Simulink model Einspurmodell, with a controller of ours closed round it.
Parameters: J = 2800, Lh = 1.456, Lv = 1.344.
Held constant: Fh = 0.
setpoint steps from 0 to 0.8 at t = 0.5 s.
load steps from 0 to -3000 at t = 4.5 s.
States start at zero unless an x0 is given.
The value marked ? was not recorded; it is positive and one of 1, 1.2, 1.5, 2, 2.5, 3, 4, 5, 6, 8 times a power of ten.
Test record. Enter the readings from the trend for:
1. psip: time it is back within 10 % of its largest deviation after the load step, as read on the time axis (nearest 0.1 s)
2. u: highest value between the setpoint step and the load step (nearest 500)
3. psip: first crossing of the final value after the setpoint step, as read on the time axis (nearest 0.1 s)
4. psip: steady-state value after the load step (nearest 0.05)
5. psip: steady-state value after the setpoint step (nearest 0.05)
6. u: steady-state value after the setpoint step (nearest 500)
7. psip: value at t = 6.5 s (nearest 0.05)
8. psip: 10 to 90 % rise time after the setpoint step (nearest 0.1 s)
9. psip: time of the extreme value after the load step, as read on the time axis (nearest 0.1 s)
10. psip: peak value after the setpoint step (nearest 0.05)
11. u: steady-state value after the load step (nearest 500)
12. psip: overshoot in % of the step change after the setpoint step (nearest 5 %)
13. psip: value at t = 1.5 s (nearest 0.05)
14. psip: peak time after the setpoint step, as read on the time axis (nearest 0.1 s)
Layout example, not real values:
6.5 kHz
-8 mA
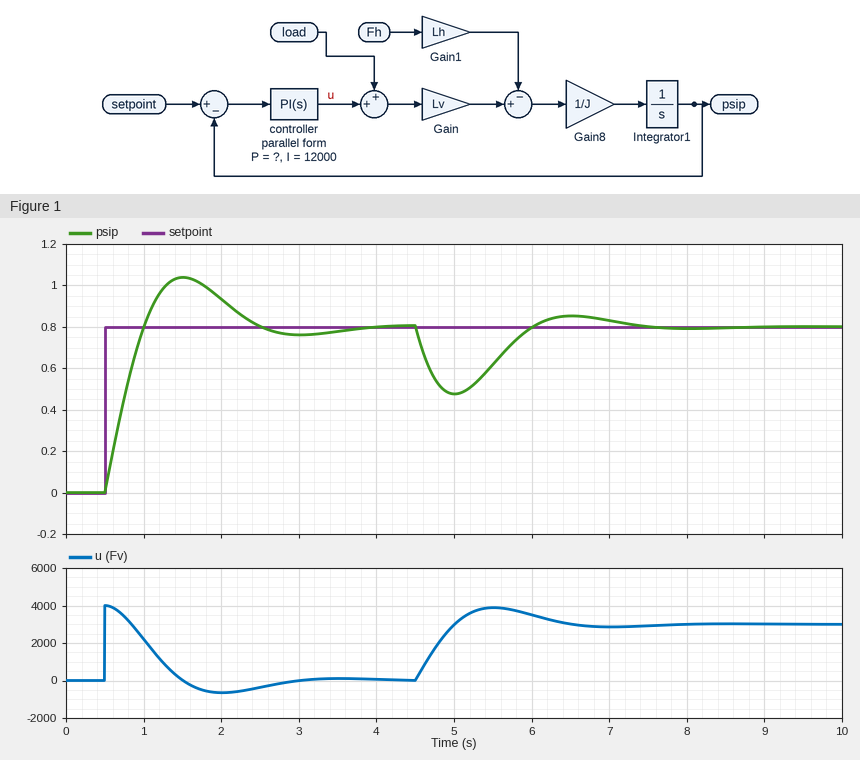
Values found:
7.0 s
4000
1.0 s
0.80
0.80
0
0.85
0.4 s
5.0 s
1.05
3000
30 %
1.05
1.5 s
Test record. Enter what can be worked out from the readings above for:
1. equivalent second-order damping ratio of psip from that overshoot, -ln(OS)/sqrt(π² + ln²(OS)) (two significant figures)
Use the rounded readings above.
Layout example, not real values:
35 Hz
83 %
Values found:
0.36
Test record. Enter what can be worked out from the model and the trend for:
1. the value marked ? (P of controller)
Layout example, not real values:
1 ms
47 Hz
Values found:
5000
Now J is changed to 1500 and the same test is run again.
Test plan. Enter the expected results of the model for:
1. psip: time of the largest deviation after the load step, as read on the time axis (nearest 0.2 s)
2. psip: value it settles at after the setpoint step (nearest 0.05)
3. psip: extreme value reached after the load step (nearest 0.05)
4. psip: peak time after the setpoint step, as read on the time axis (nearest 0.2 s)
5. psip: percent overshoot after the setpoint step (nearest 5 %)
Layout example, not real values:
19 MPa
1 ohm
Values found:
4.8 s
0.80
0.40
1.2 s
20 %
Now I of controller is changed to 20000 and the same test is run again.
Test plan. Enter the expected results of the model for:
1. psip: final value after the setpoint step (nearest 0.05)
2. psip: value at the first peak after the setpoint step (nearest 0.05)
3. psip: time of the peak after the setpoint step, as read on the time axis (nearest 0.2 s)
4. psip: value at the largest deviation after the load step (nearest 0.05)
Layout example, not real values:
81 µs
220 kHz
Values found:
0.80
1.10
1.4 s
0.50
